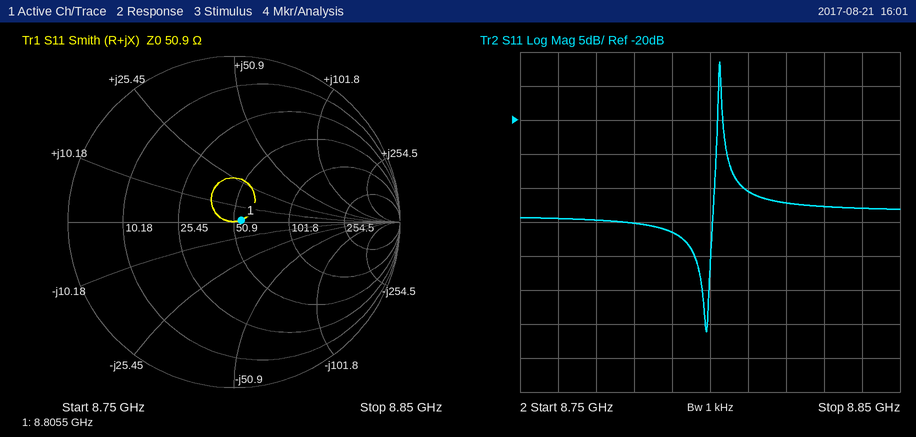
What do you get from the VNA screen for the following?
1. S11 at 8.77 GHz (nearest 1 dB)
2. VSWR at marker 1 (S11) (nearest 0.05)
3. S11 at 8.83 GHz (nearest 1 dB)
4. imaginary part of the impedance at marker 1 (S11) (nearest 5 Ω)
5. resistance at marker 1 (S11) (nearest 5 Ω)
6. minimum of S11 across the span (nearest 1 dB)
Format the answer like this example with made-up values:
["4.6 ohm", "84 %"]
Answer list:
["-35 dB", "1.10", "-33 dB", "0 Ω", "55 Ω", "-51 dB"]
